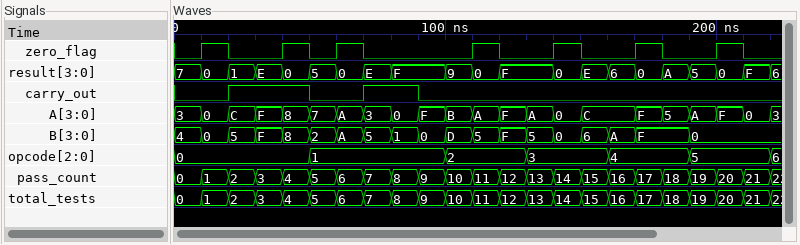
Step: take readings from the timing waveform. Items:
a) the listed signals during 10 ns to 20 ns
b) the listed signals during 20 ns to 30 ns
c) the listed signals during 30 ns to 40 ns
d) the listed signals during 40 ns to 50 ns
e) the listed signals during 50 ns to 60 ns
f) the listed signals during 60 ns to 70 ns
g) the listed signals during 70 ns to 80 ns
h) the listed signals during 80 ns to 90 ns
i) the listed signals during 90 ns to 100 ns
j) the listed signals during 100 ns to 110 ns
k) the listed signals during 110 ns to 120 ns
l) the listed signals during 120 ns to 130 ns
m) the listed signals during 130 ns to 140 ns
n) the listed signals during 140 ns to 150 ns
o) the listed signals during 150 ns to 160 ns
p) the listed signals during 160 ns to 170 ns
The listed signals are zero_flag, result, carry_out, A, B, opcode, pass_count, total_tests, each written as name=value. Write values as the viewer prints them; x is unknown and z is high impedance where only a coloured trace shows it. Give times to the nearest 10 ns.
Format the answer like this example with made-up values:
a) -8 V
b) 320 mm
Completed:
a) zero_flag=1, result=0, carry_out=0, A=0, B=0, opcode=0, pass_count=1, total_tests=1
b) zero_flag=0, result=1, carry_out=1, A=C, B=5, opcode=0, pass_count=2, total_tests=2
c) zero_flag=0, result=E, carry_out=1, A=F, B=F, opcode=0, pass_count=3, total_tests=3
d) zero_flag=1, result=0, carry_out=1, A=8, B=8, opcode=0, pass_count=4, total_tests=4
e) zero_flag=0, result=5, carry_out=0, A=7, B=2, opcode=1, pass_count=5, total_tests=5
f) zero_flag=1, result=0, carry_out=0, A=A, B=A, opcode=1, pass_count=6, total_tests=6
g) zero_flag=0, result=E, carry_out=1, A=3, B=5, opcode=1, pass_count=7, total_tests=7
h) zero_flag=0, result=F, carry_out=1, A=0, B=1, opcode=1, pass_count=8, total_tests=8
i) zero_flag=0, result=F, carry_out=0, A=F, B=0, opcode=1, pass_count=9, total_tests=9
j) zero_flag=0, result=9, carry_out=0, A=B, B=D, opcode=2, pass_count=10, total_tests=10
k) zero_flag=1, result=0, carry_out=0, A=A, B=5, opcode=2, pass_count=11, total_tests=11
l) zero_flag=0, result=F, carry_out=0, A=F, B=F, opcode=2, pass_count=12, total_tests=12
m) zero_flag=0, result=F, carry_out=0, A=A, B=5, opcode=3, pass_count=13, total_tests=13
n) zero_flag=1, result=0, carry_out=0, A=0, B=0, opcode=3, pass_count=14, total_tests=14
o) zero_flag=0, result=E, carry_out=0, A=C, B=6, opcode=3, pass_count=15, total_tests=15
p) zero_flag=0, result=6, carry_out=0, A=C, B=A, opcode=4, pass_count=16, total_tests=16
